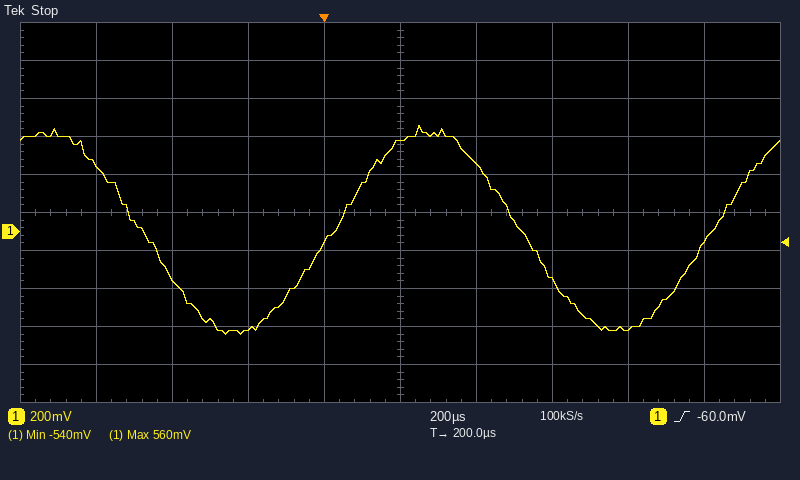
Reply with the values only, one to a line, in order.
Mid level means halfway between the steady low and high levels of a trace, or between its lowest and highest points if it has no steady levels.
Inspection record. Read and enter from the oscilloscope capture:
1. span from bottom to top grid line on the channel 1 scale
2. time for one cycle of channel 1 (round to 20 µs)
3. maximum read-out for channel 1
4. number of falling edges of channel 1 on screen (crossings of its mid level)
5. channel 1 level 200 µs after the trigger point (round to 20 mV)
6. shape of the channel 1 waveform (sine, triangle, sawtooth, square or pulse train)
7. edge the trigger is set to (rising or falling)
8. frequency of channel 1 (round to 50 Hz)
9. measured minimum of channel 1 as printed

2 V
1.00 ms
560 mV
2
480 mV
sine
rising
1.00 kHz
-540 mV
